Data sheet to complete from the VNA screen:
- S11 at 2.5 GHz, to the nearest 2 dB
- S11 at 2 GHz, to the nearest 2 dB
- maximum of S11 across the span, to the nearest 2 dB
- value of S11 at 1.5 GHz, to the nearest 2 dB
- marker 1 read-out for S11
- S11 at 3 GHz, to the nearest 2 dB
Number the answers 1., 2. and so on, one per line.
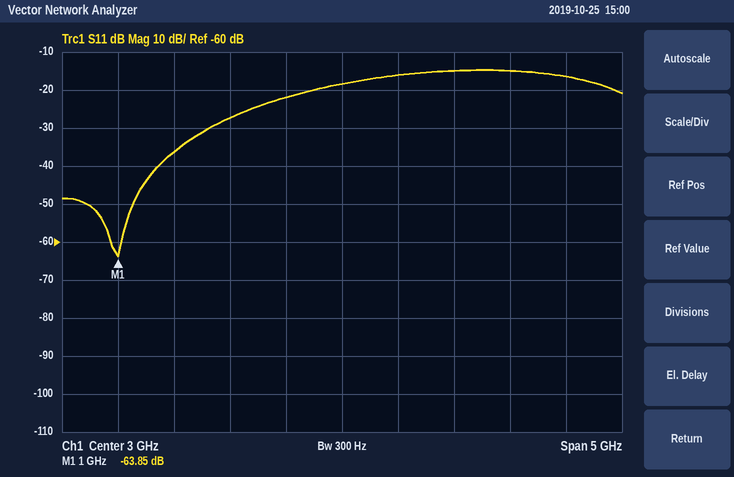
1. -22 dB
2. -28 dB
3. -14 dB
4. -36 dB
5. -63.85 dB
6. -18 dB
